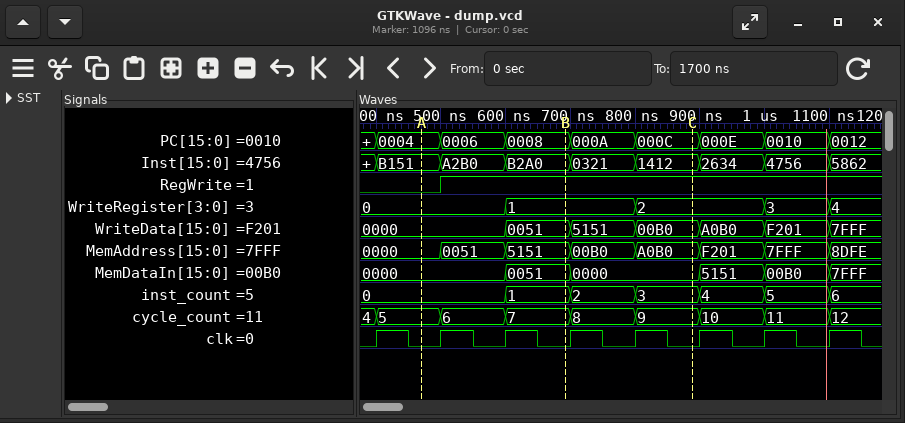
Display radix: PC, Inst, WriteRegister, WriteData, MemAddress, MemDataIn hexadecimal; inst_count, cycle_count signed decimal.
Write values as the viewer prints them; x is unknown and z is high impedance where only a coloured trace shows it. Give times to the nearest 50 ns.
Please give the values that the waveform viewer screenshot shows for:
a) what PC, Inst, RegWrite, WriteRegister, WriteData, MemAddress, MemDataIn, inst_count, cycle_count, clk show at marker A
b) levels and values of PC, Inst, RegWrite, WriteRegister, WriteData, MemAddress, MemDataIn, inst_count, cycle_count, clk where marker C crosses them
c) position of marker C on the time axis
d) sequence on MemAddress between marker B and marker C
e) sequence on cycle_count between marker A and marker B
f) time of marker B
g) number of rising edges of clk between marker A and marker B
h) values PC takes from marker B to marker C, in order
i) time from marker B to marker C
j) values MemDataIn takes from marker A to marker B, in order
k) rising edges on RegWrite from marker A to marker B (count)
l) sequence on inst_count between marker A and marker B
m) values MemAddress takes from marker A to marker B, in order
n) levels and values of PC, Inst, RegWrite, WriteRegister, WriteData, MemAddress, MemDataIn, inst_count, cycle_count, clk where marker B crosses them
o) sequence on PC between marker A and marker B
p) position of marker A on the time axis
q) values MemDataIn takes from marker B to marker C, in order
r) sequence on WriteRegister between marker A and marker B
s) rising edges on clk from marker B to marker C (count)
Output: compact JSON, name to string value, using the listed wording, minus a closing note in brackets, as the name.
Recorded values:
{"what PC, Inst, RegWrite, WriteRegister, WriteData, MemAddress, MemDataIn, inst_count, cycle_count, clk show at marker A": "PC=0004, Inst=B151, RegWrite=0, WriteRegister=0, WriteData=0000, MemAddress=0000, MemDataIn=0000, inst_count=0, cycle_count=5, clk=0", "levels and values of PC, Inst, RegWrite, WriteRegister, WriteData, MemAddress, MemDataIn, inst_count, cycle_count, clk where marker C crosses them": "PC=000C, Inst=1412, RegWrite=1, WriteRegister=2, WriteData=00B0, MemAddress=A0B0, MemDataIn=0000, inst_count=3, cycle_count=9, clk=0", "position of marker C on the time axis": "900 ns", "sequence on MemAddress between marker B and marker C": "5151, 00B0, A0B0", "sequence on cycle_count between marker A and marker B": "5, 6, 7", "time of marker B": "700 ns", "number of rising edges of clk between marker A and marker B": "2", "values PC takes from marker B to marker C, in order": "0008, 000A, 000C", "time from marker B to marker C": "200 ns", "values MemDataIn takes from marker A to marker B, in order": "0000, 0051", "rising edges on RegWrite from marker A to marker B": "1", "sequence on inst_count between marker A and marker B": "0, 1", "values MemAddress takes from marker A to marker B, in order": "0000, 0051, 5151", "levels and values of PC, Inst, RegWrite, WriteRegister, WriteData, MemAddress, MemDataIn, inst_count, cycle_count, clk where marker B crosses them": "PC=0008, Inst=B2A0, RegWrite=1, WriteRegister=1, WriteData=0051, MemAddress=5151, MemDataIn=0051, inst_count=1, cycle_count=7, clk=0", "sequence on PC between marker A and marker B": "0004, 0006, 0008", "position of marker A on the time axis": "450 ns", "values MemDataIn takes from marker B to marker C, in order": "0051, 0000", "sequence on WriteRegister between marker A and marker B": "0, 1", "rising edges on clk from marker B to marker C": "2"}
